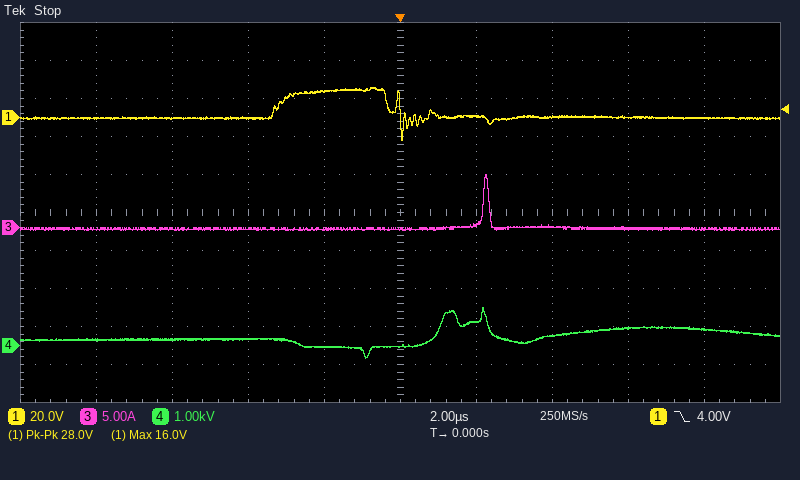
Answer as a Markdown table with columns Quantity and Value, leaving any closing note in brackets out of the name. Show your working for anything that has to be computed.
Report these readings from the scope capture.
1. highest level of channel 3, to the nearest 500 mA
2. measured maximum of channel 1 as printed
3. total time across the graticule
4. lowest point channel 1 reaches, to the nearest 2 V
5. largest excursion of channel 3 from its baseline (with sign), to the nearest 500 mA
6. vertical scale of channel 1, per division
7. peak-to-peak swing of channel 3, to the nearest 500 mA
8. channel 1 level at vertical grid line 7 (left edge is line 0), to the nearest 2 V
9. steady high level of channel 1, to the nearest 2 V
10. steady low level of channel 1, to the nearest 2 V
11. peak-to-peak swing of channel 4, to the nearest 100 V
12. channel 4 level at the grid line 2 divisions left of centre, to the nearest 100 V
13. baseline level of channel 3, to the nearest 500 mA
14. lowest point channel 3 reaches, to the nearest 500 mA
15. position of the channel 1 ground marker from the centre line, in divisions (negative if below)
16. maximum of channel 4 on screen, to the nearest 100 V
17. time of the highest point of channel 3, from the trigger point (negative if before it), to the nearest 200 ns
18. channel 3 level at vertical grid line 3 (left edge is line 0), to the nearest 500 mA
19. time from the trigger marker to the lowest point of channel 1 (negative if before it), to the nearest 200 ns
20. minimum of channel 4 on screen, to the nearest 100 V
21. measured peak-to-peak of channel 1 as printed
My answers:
| Quantity | Value |
|---|---|
| highest level of channel 3, to the nearest 500 mA | 7.0 A |
| measured maximum of channel 1 as printed | 16.0 V |
| total time across the graticule | 20 µs |
| lowest point channel 1 reaches, to the nearest 2 V | -12 V |
| largest excursion of channel 3 from its baseline (with sign), to the nearest 500 mA | 7.0 A − (0.0 A) = +7.0 A |
| vertical scale of channel 1, per division | 20 V |
| peak-to-peak swing of channel 3, to the nearest 500 mA | 7.0 A − (-500 mA) = 7.5 A |
| channel 1 level at vertical grid line 7 (left edge is line 0), to the nearest 2 V | 0 V |
| steady high level of channel 1, to the nearest 2 V | 14 V |
| steady low level of channel 1, to the nearest 2 V | 0 V |
| peak-to-peak swing of channel 4, to the nearest 100 V | 1.0 kV − (-300 V) = 1.3 kV |
| channel 4 level at the grid line 2 divisions left of centre, to the nearest 100 V | 200 V |
| baseline level of channel 3, to the nearest 500 mA | 0.0 A |
| lowest point channel 3 reaches, to the nearest 500 mA | -500 mA |
| position of the channel 1 ground marker from the centre line, in divisions | +2.5 div |
| maximum of channel 4 on screen, to the nearest 100 V | 1.0 kV |
| time of the highest point of channel 3, from the trigger point (negative if before it), to the nearest 200 ns | +2.2 µs |
| channel 3 level at vertical grid line 3 (left edge is line 0), to the nearest 500 mA | 0.0 A |
| time from the trigger marker to the lowest point of channel 1 (negative if before it), to the nearest 200 ns | 0.0 µs |
| minimum of channel 4 on screen, to the nearest 100 V | -300 V |
| measured peak-to-peak of channel 1 as printed | 28.0 V |
